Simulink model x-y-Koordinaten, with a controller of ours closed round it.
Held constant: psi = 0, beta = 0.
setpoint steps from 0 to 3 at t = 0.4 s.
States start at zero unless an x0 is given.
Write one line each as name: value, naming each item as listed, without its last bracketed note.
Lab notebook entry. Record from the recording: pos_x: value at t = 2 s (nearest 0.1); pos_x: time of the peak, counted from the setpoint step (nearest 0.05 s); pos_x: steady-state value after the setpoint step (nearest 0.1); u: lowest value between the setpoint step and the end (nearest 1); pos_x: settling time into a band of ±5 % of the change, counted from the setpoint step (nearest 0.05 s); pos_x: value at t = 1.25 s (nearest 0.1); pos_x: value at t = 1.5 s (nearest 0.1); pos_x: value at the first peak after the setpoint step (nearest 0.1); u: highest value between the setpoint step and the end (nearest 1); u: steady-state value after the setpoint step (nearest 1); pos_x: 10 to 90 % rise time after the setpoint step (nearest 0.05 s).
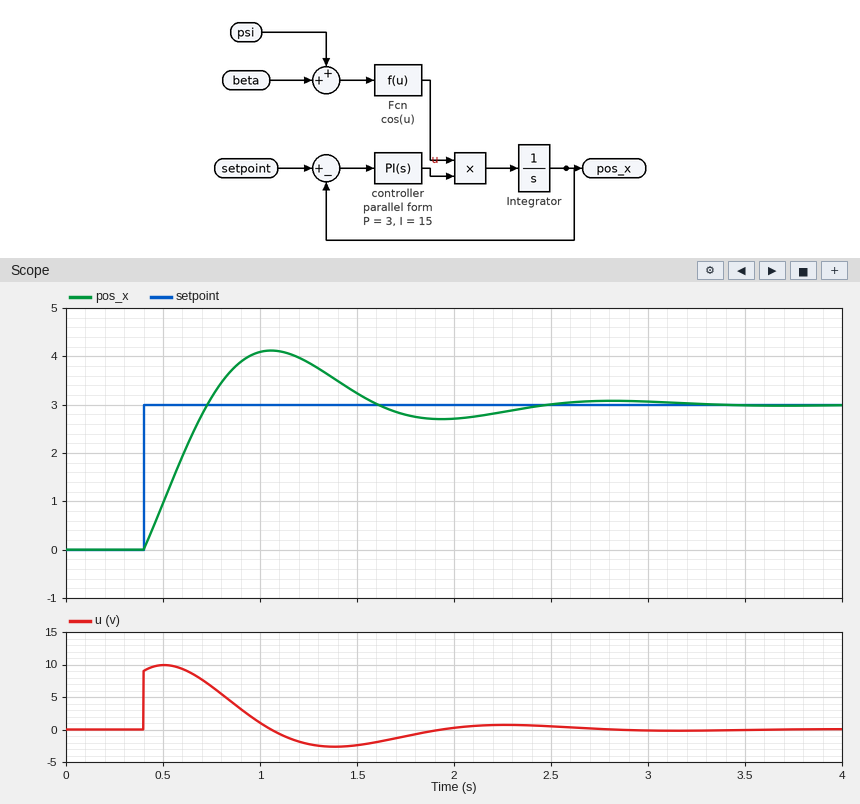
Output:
pos_x: value at t = 2 s: 2.7
pos_x: time of the peak, counted from the setpoint step: 0.65 s
pos_x: steady-state value after the setpoint step: 3.0
u: lowest value between the setpoint step and the end: -3
pos_x: settling time into a band of ±5 % of the change, counted from the setpoint step: 1.85 s
pos_x: value at t = 1.25 s: 3.9
pos_x: value at t = 1.5 s: 3.2
pos_x: value at the first peak after the setpoint step: 4.1
u: highest value between the setpoint step and the end: 10
u: steady-state value after the setpoint step: 0
pos_x: 10 to 90 % rise time after the setpoint step: 0.25 s
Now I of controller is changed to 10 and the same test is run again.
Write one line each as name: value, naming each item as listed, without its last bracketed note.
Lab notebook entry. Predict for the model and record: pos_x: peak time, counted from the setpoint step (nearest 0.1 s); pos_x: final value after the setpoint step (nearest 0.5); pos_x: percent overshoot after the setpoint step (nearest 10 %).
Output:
pos_x: peak time, counted from the setpoint step: 0.8 s
pos_x: final value after the setpoint step: 3.0
pos_x: percent overshoot after the setpoint step: 30 %
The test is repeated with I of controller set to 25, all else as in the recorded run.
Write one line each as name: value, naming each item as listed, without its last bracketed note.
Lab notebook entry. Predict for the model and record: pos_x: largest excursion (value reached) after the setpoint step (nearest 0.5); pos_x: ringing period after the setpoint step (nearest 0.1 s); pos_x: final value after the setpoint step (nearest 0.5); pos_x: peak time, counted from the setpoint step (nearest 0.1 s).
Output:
pos_x: largest excursion (value reached) after the setpoint step: 4.5
pos_x: ringing period after the setpoint step: 1.3 s
pos_x: final value after the setpoint step: 3.0
pos_x: peak time, counted from the setpoint step: 0.5 s
